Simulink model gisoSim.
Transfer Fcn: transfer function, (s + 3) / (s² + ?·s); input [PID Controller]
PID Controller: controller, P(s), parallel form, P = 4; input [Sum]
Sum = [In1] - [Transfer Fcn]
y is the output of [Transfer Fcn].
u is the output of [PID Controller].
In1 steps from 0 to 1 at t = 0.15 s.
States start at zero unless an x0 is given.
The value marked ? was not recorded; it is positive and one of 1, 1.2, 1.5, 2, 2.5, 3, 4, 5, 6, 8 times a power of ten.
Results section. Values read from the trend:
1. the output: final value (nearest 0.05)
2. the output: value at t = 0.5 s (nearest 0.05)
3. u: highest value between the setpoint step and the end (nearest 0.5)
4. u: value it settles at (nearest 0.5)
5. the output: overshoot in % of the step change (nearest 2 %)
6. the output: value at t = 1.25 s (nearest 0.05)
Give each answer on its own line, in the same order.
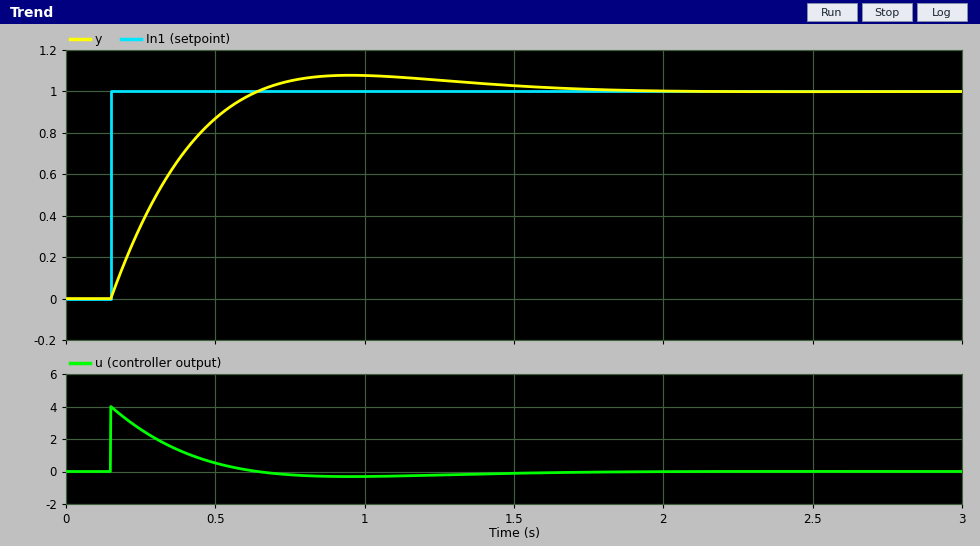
1.00
0.85
4.0
0.0
8 %
1.05
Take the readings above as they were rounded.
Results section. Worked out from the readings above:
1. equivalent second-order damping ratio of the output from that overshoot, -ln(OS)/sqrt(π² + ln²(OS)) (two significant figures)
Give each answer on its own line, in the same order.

0.63
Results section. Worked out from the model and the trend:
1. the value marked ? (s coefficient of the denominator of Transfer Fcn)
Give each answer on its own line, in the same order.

1.5
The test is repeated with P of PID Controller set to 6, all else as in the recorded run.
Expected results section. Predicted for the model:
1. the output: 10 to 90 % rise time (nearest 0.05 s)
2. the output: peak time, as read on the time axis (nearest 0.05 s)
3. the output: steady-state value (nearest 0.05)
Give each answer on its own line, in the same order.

0.25 s
0.75 s
1.00
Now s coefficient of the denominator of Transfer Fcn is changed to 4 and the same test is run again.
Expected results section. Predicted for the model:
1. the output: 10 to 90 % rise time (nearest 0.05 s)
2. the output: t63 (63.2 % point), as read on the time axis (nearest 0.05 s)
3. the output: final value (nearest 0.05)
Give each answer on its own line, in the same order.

0.80 s
0.45 s
1.00
